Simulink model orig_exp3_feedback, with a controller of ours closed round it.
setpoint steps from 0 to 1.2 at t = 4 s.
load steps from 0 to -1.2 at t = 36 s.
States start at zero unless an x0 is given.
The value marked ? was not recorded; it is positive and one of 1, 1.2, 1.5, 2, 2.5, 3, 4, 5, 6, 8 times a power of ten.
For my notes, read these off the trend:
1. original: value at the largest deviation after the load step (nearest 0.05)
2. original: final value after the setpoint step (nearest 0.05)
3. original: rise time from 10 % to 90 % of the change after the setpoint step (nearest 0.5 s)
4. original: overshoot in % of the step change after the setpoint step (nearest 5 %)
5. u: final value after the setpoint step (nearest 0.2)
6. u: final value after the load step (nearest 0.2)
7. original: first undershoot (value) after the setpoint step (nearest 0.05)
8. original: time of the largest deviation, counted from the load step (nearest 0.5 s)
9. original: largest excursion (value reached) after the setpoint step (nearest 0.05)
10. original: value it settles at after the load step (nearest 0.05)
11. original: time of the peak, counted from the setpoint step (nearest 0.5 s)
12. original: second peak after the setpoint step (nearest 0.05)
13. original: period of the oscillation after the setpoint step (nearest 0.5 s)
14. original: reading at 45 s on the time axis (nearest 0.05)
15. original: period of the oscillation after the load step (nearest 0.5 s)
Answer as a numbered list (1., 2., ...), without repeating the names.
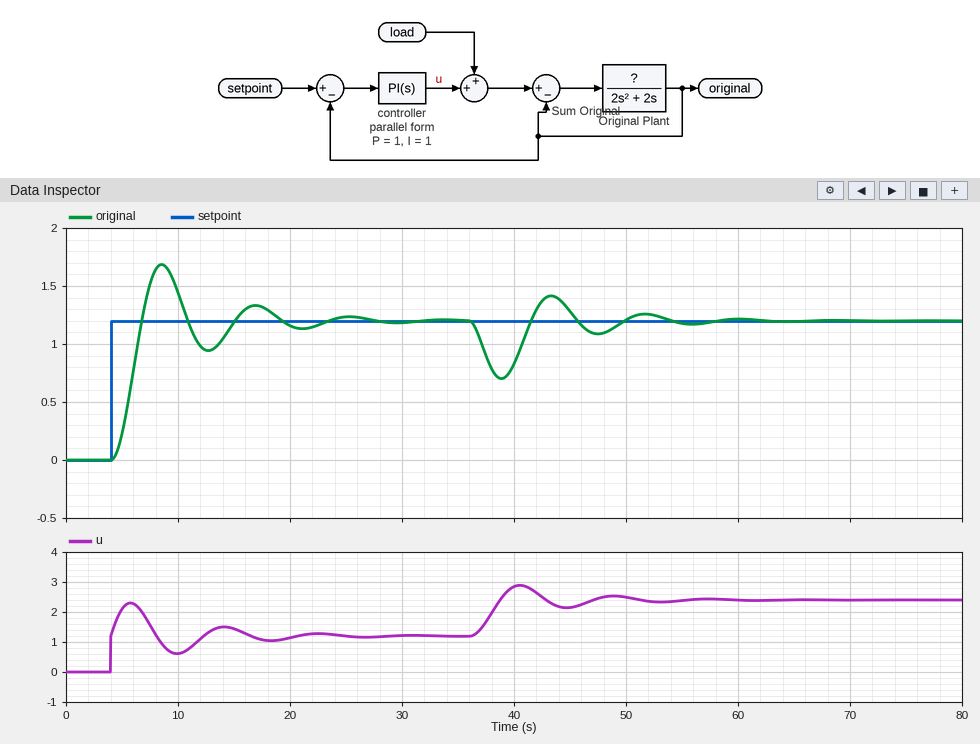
1. 0.70
2. 1.20
3. 2.0 s
4. 40 %
5. 1.2
6. 2.4
7. 0.95
8. 3.0 s
9. 1.70
10. 1.20
11. 4.5 s
12. 1.35
13. 8.5 s
14. 1.30
15. 8.5 s
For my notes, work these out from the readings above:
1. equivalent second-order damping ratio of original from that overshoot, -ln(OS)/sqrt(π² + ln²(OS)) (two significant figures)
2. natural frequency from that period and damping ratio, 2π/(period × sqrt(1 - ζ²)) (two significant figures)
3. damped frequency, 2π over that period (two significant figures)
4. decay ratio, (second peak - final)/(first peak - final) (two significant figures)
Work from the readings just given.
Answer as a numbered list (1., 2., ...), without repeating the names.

1. 0.28
2. 0.77 rad/s
3. 0.74 rad/s
4. 0.30
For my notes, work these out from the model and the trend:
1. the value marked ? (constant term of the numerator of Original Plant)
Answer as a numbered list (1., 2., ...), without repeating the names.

1. 0.8
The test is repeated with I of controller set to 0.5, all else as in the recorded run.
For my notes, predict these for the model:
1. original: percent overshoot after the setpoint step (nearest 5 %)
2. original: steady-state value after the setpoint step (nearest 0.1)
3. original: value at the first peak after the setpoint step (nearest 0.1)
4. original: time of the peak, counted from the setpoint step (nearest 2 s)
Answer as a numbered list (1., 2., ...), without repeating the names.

1. 10 %
2. 1.2
3. 1.3
4. 6 s
